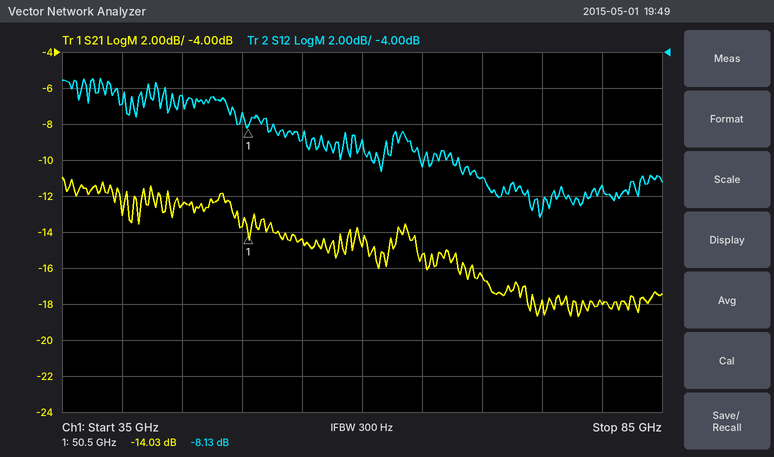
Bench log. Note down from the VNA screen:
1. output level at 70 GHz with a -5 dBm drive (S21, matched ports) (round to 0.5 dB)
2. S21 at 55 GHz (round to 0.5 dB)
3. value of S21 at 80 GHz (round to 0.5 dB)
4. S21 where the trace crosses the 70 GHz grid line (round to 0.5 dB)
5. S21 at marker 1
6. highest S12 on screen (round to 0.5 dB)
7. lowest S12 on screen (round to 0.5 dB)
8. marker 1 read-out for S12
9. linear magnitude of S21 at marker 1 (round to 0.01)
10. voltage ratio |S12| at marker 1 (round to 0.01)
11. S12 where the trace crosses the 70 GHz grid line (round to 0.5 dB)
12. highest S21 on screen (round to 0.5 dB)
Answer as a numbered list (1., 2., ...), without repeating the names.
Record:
1. -21.5 dBm
2. -14.5 dB
3. -18.0 dB
4. -16.5 dB
5. -14.03 dB
6. -5.5 dB
7. -13.0 dB
8. -8.13 dB
9. 0.20
10. 0.39
11. -11.0 dB
12. -11.0 dB
